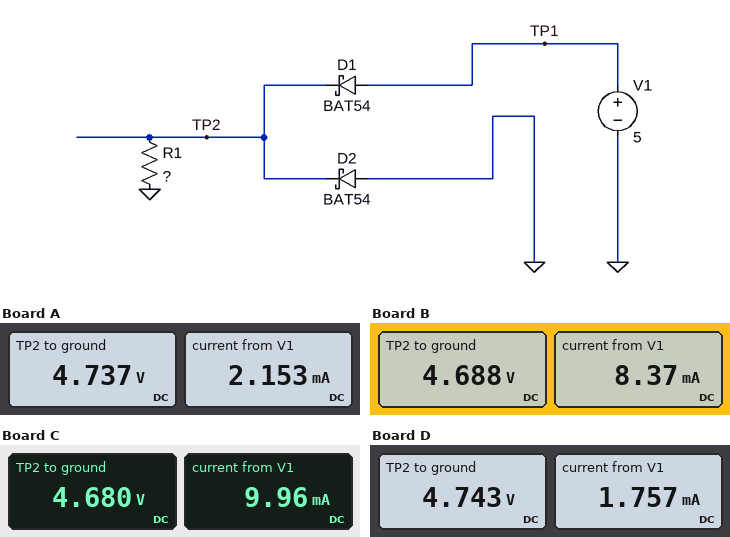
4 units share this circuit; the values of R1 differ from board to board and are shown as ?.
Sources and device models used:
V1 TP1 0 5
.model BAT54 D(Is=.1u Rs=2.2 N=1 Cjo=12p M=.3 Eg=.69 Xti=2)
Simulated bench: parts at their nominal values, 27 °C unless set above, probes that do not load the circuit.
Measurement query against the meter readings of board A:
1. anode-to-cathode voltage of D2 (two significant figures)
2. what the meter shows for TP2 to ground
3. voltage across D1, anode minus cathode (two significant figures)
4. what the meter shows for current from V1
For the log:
-4.7 V
4.737 V
260 mV
2.153 mA
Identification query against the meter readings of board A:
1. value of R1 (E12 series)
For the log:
2.2 kΩ
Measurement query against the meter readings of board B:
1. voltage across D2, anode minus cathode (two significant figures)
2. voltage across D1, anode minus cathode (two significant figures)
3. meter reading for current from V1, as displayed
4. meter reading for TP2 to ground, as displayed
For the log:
-4.7 V
310 mV
8.37 mA
4.688 V
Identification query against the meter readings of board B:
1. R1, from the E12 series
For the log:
560 Ω
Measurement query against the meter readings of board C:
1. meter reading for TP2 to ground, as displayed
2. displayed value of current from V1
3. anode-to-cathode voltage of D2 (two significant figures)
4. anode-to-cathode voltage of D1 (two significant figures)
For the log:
4.680 V
9.96 mA
-4.7 V
320 mV
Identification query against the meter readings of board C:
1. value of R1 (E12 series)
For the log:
470 Ω
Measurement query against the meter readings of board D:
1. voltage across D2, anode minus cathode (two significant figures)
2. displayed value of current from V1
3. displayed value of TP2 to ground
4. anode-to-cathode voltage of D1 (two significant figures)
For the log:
-4.7 V
1.757 mA
4.743 V
260 mV
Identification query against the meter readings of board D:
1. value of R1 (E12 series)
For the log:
2.7 kΩ
